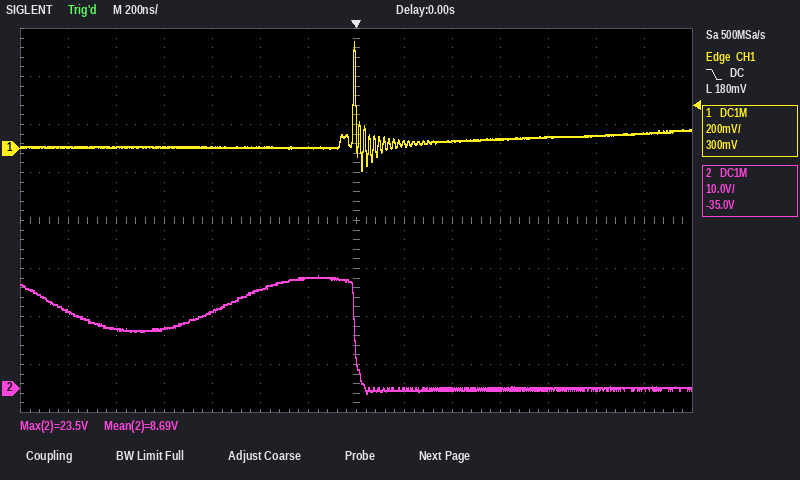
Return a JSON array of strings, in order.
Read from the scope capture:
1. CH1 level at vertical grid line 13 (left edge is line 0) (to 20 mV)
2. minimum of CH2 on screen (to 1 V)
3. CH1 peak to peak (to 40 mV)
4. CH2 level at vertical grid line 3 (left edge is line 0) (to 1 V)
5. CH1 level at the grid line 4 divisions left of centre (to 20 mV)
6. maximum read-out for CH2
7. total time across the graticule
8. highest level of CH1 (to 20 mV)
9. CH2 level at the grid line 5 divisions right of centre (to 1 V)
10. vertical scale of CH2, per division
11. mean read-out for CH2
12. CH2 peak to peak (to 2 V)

["60 mV", "-1 V", "520 mV", "13 V", "0 mV", "23.5 V", "2.8 µs", "440 mV", "0 V", "10 V", "8.69 V", "24 V"]
